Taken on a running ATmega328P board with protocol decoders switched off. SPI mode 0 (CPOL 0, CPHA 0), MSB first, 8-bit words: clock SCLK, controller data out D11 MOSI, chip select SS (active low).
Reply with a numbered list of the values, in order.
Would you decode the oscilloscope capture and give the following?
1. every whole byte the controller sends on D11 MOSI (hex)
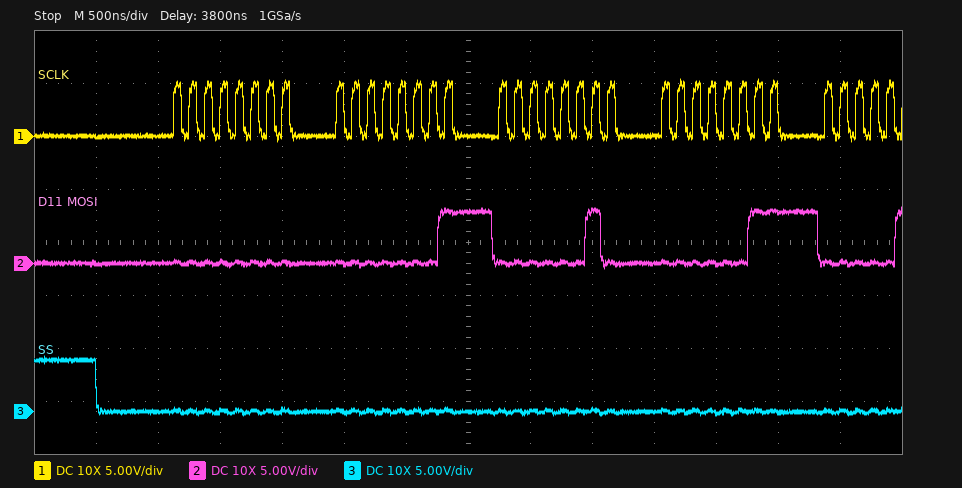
1. 00 01 02 03
